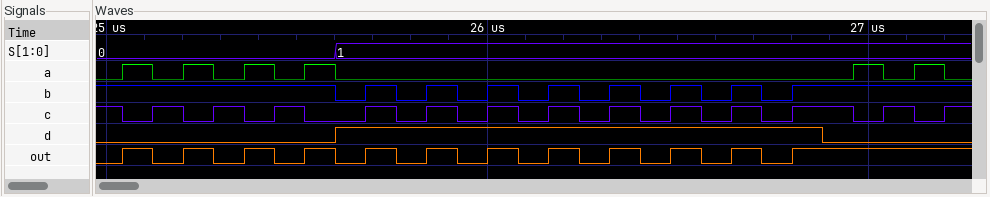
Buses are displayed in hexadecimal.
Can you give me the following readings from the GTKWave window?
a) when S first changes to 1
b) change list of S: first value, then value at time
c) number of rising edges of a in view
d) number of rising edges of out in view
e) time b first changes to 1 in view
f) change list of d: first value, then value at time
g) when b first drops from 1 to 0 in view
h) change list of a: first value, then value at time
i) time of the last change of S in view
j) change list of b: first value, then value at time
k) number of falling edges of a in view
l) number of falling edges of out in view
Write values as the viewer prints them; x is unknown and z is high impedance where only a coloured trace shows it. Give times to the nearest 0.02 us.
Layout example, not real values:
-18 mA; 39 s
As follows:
25.6 us; 0, 1 at 25.6 us; 6; 12; 25.68 us; 0, 1 at 25.6 us, 0 at 26.88 us; 25.6 us; 0, 1 at 25.04 us, 0 at 25.12 us, 1 at 25.2 us, 0 at 25.28 us, 1 at 25.36 us, 0 at 25.44 us, 1 at 25.52 us, 0 at 25.6 us, 1 at 26.96 us, 0 at 27.04 us, 1 at 27.12 us, 0 at 27.2 us; 25.6 us; 1, 0 at 25.6 us, 1 at 25.68 us, 0 at 25.76 us, 1 at 25.84 us, 0 at 25.92 us, 1 at 26 us, 0 at 26.08 us, 1 at 26.16 us, 0 at 26.24 us, 1 at 26.32 us, 0 at 26.4 us, 1 at 26.48 us, 0 at 26.56 us, 1 at 26.64 us, 0 at 26.72 us, 1 at 26.8 us; 6; 11
